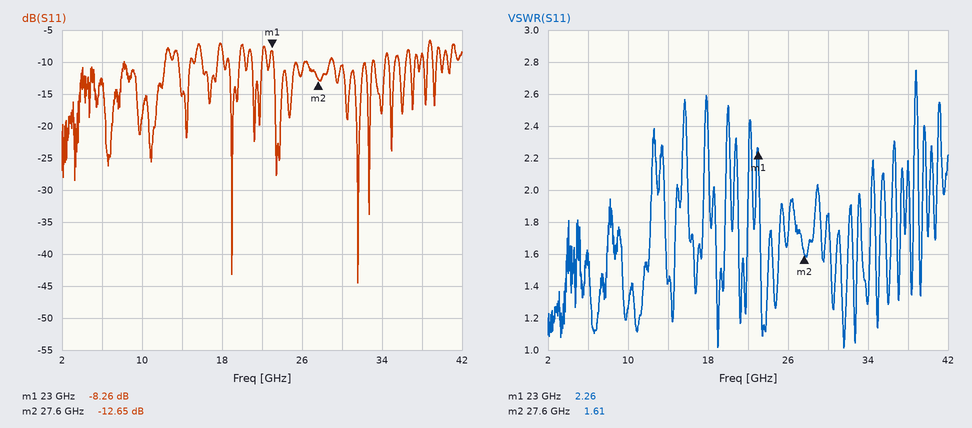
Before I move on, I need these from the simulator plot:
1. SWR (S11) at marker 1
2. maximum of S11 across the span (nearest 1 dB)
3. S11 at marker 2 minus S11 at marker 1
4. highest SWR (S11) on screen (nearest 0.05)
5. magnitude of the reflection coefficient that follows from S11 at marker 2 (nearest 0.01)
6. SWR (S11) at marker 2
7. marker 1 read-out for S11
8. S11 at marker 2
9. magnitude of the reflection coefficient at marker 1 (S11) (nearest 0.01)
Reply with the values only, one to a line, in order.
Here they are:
2.26
-7 dB
-4.39 dB
2.75
0.23
1.61
-8.26 dB
-12.65 dB
0.39
